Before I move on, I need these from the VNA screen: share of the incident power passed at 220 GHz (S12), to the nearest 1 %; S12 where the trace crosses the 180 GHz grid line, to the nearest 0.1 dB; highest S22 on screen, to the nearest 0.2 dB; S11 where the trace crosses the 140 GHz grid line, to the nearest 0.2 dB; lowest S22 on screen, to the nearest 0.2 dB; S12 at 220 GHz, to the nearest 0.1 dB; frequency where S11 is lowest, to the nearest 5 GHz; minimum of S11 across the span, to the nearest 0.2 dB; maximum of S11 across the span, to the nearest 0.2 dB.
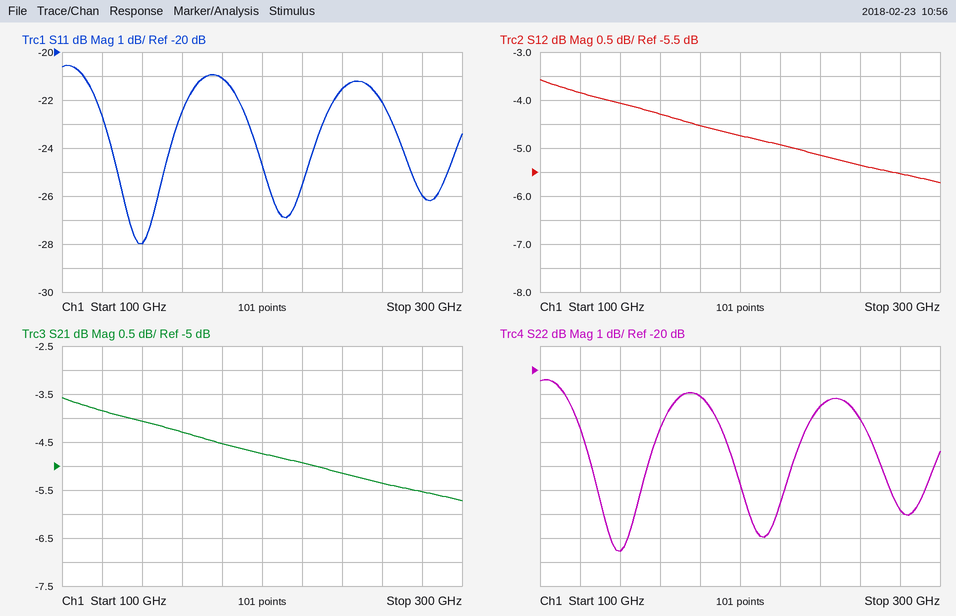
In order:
32 %
-4.5 dB
-20.4 dB
-28.0 dB
-27.6 dB
-4.9 dB
140 GHz
-28.0 dB
-20.6 dB
